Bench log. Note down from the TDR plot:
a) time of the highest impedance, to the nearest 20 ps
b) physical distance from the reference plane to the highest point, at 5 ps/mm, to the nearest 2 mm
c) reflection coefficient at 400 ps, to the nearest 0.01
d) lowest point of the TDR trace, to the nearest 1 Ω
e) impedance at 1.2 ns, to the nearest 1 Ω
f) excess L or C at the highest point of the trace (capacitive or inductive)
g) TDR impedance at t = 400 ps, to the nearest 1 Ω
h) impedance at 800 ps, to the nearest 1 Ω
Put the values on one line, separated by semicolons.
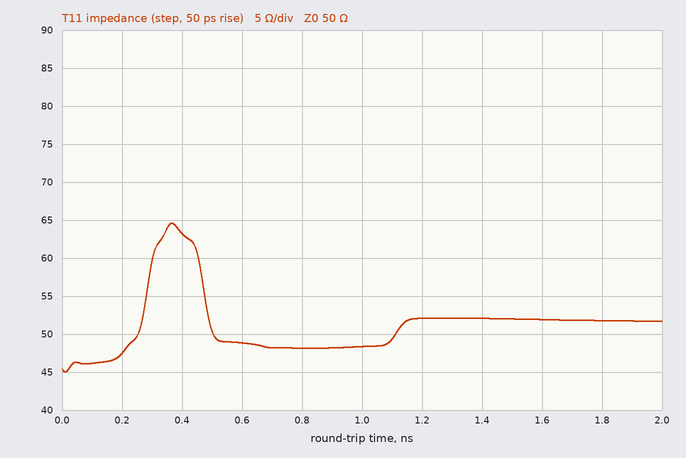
360 ps; 36 mm; +0.12; 45 Ω; 52 Ω; inductive; 63 Ω; 48 Ω
